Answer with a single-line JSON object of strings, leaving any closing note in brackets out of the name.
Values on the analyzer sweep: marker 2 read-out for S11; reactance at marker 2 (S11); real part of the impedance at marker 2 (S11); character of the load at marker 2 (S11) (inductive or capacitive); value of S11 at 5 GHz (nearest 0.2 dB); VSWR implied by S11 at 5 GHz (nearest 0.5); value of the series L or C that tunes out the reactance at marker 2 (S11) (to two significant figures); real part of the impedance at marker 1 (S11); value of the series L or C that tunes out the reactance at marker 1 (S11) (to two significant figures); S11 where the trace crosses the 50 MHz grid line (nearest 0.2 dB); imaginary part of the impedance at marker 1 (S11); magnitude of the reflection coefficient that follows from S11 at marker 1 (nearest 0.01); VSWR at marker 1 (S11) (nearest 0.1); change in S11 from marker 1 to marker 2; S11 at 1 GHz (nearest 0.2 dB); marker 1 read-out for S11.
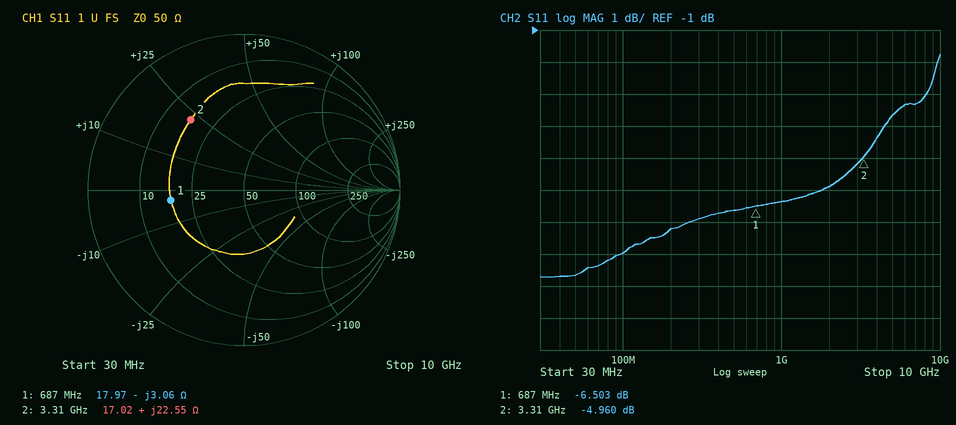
{"marker 2 read-out for S11": "-4.960 dB", "reactance at marker 2": "+22.55 Ω", "real part of the impedance at marker 2": "17.02 Ω", "character of the load at marker 2 (S11)": "inductive", "value of S11 at 5 GHz": "-3.6 dB", "VSWR implied by S11 at 5 GHz": "5.0", "value of the series L or C that tunes out the reactance at marker 2 (S11)": "2.1 pF", "real part of the impedance at marker 1": "17.97 Ω", "value of the series L or C that tunes out the reactance at marker 1 (S11)": "710 pH", "S11 where the trace crosses the 50 MHz grid line": "-8.6 dB", "imaginary part of the impedance at marker 1": "-3.06 Ω", "magnitude of the reflection coefficient that follows from S11 at marker 1": "0.47", "VSWR at marker 1 (S11)": "2.8", "change in S11 from marker 1 to marker 2": "1.543 dB", "S11 at 1 GHz": "-6.4 dB", "marker 1 read-out for S11": "-6.503 dB"}
